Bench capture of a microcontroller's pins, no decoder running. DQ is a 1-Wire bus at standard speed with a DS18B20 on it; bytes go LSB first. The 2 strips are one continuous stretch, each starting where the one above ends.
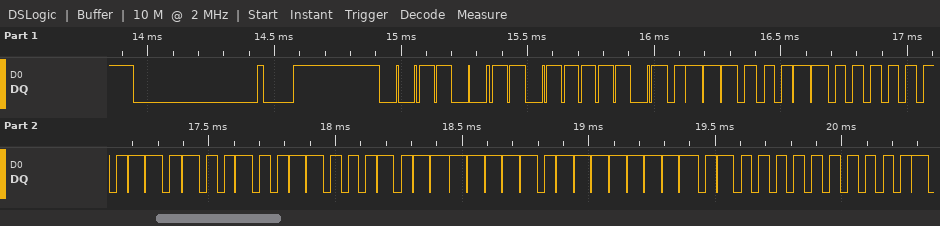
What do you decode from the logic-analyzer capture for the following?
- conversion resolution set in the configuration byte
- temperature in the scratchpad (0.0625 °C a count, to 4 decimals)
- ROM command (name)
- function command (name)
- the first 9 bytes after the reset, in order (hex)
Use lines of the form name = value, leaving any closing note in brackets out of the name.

conversion resolution set in the configuration byte = 12 bits
temperature in the scratchpad = 24.8750 °C
ROM command = Skip ROM
function command = Read Scratchpad
the first 9 bytes after the reset, in order = CC BE 8E 01 4B 46 7F FF 02
